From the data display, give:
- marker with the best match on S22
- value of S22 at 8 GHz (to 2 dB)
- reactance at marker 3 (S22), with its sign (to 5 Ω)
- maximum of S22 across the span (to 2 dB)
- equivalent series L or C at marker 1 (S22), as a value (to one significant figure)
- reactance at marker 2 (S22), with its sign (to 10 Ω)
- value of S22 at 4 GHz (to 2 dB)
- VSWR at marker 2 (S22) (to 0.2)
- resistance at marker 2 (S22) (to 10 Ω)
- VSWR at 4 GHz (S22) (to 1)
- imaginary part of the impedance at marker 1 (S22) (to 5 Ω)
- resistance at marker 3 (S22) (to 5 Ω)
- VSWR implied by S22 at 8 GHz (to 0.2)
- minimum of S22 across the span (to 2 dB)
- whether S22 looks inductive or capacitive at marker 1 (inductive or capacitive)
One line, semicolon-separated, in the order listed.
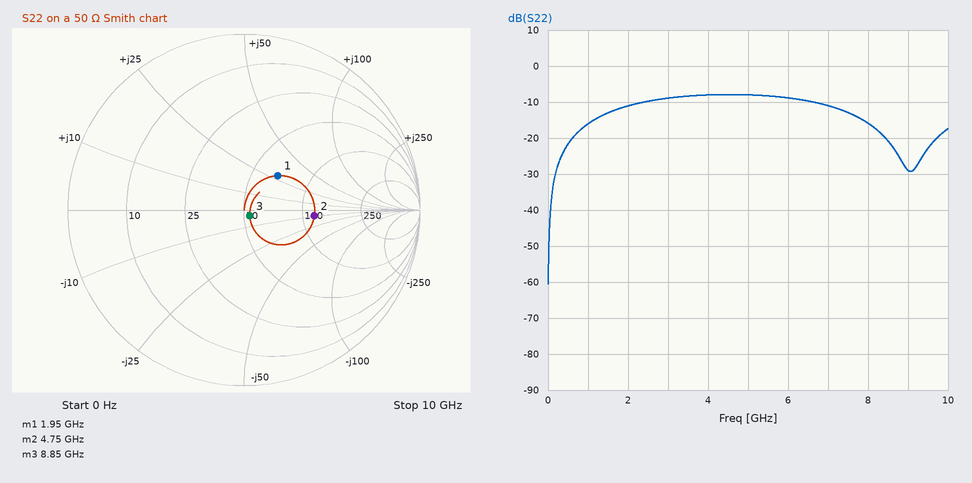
marker 3; -16 dB; -5 Ω; -8 dB; 2 nH; -10 Ω; -8 dB; 2.4; 120 Ω; 2; +30 Ω; 55 Ω; 1.4; -60 dB; inductive
